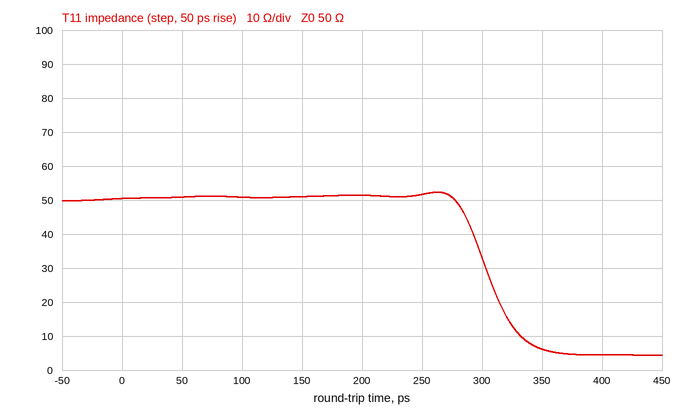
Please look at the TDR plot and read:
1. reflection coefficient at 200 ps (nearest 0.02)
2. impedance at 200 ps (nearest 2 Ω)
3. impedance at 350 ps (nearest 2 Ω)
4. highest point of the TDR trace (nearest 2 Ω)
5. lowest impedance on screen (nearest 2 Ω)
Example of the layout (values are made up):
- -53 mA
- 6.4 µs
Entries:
- +0.02
- 52 Ω
- 6 Ω
- 52 Ω
- 4 Ω
